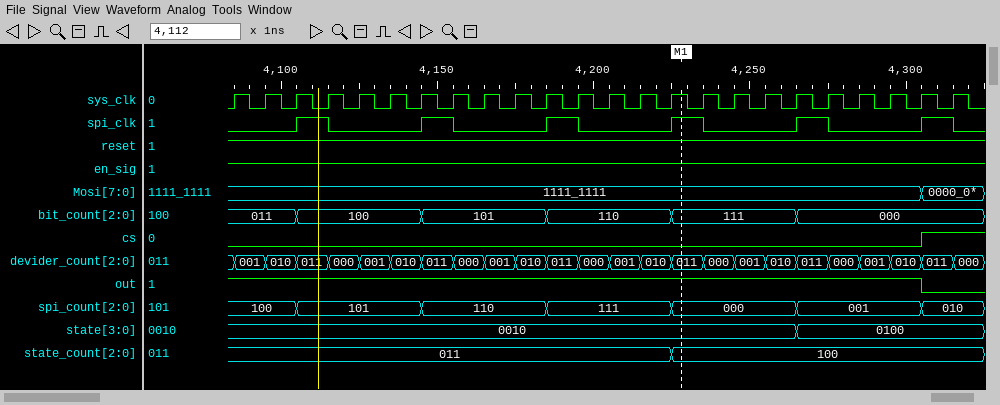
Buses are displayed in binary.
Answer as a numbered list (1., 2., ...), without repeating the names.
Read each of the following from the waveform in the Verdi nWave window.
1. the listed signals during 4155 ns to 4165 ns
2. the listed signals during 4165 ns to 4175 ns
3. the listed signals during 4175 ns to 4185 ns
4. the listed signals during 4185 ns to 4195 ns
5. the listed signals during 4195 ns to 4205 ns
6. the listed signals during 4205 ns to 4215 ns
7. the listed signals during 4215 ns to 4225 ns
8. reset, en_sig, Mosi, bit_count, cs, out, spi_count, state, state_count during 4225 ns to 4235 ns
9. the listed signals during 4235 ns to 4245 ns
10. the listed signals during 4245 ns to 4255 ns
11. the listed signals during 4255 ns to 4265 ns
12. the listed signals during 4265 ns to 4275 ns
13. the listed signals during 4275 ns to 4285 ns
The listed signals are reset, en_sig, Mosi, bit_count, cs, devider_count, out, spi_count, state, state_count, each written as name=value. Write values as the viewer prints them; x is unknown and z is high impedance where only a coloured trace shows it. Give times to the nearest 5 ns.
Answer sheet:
1. reset=1, en_sig=1, Mosi=1111_1111, bit_count=101, cs=0, devider_count=000, out=1, spi_count=110, state=0010, state_count=011
2. reset=1, en_sig=1, Mosi=1111_1111, bit_count=101, cs=0, devider_count=001, out=1, spi_count=110, state=0010, state_count=011
3. reset=1, en_sig=1, Mosi=1111_1111, bit_count=101, cs=0, devider_count=010, out=1, spi_count=110, state=0010, state_count=011
4. reset=1, en_sig=1, Mosi=1111_1111, bit_count=110, cs=0, devider_count=011, out=1, spi_count=111, state=0010, state_count=011
5. reset=1, en_sig=1, Mosi=1111_1111, bit_count=110, cs=0, devider_count=000, out=1, spi_count=111, state=0010, state_count=011
6. reset=1, en_sig=1, Mosi=1111_1111, bit_count=110, cs=0, devider_count=001, out=1, spi_count=111, state=0010, state_count=011
7. reset=1, en_sig=1, Mosi=1111_1111, bit_count=110, cs=0, devider_count=010, out=1, spi_count=111, state=0010, state_count=011
8. reset=1, en_sig=1, Mosi=1111_1111, bit_count=111, cs=0, out=1, spi_count=000, state=0010, state_count=100
9. reset=1, en_sig=1, Mosi=1111_1111, bit_count=111, cs=0, devider_count=000, out=1, spi_count=000, state=0010, state_count=100
10. reset=1, en_sig=1, Mosi=1111_1111, bit_count=111, cs=0, devider_count=001, out=1, spi_count=000, state=0010, state_count=100
11. reset=1, en_sig=1, Mosi=1111_1111, bit_count=111, cs=0, devider_count=010, out=1, spi_count=000, state=0010, state_count=100
12. reset=1, en_sig=1, Mosi=1111_1111, bit_count=000, cs=0, devider_count=011, out=1, spi_count=001, state=0100, state_count=100
13. reset=1, en_sig=1, Mosi=1111_1111, bit_count=000, cs=0, devider_count=000, out=1, spi_count=001, state=0100, state_count=100
